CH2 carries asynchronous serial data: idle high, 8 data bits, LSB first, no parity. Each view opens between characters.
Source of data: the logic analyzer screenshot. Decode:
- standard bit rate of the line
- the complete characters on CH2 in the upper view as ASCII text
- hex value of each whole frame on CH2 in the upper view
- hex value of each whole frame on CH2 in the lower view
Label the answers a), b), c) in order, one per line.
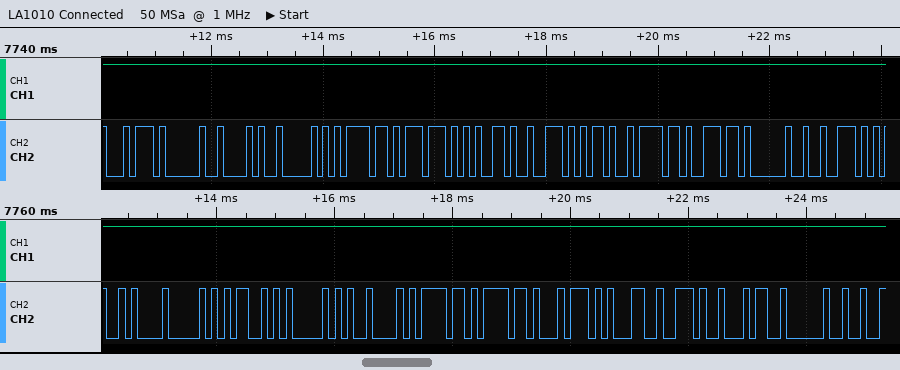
a) 9600 baud
b) "t (Power-on r"
c) 74, 20, 28, 50, 6F, 77, 65, 72, 2D, 6F, 6E, 20, 72
d) 0A, 50, 53, 50, 42, 6F, 6F, 74, 31, 2E, 34, 20
